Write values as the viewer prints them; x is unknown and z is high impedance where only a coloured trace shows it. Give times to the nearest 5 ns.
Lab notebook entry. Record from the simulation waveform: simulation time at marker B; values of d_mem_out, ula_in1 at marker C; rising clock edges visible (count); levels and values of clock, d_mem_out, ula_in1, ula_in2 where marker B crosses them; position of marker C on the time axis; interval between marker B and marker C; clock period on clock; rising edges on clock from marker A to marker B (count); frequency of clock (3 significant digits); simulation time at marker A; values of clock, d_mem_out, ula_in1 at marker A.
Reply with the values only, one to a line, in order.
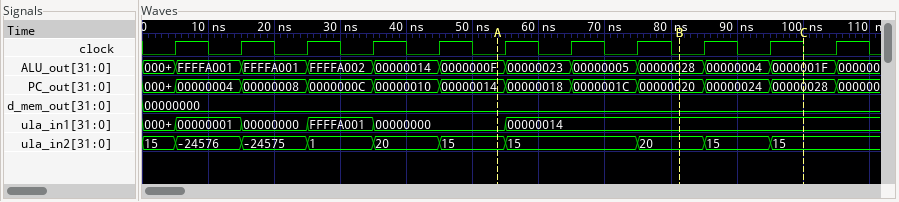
80 ns
d_mem_out=00000000, ula_in1=00000014
11
clock=0, d_mem_out=00000000, ula_in1=00000014, ula_in2=20
100 ns
20 ns
10 ns
3
100 MHz
55 ns
clock=0, d_mem_out=00000000, ula_in1=00000000
